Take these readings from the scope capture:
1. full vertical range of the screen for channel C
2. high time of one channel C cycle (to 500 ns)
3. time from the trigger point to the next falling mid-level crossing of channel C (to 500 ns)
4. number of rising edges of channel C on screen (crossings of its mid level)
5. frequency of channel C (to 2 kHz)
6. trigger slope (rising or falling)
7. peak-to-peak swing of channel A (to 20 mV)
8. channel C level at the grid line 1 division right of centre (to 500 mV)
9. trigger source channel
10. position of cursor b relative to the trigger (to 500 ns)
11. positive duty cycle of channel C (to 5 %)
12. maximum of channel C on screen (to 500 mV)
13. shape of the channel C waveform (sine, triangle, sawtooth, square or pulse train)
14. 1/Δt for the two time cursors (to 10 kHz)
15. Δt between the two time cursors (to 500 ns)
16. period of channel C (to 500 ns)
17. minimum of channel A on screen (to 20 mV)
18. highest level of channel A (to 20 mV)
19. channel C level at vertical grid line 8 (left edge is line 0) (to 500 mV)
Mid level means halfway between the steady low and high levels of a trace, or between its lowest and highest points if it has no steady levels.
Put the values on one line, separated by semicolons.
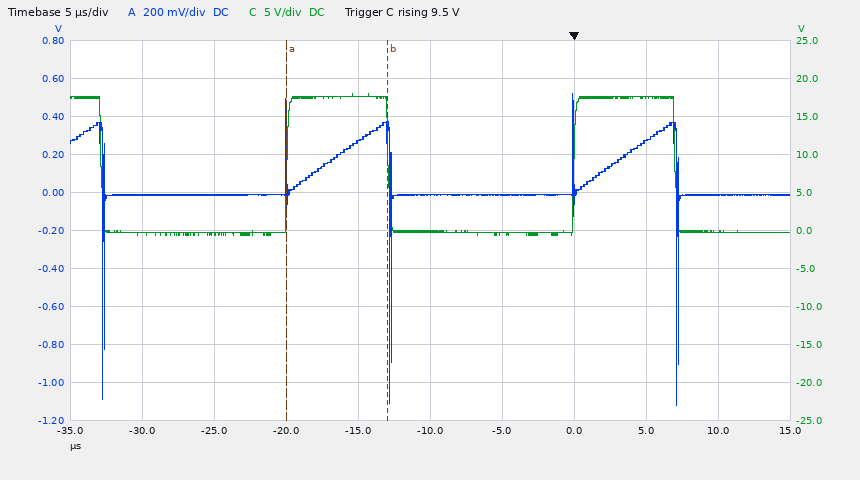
50 V; 7.0 µs; 7.0 µs; 2; 50 kHz; rising; 1.64 V; -500 mV; channel C; -13.0 µs; 35 %; 18.0 V; pulse train; 140 kHz; 7.0 µs; 20.0 µs; -1.12 V; 520 mV; 17.5 V
